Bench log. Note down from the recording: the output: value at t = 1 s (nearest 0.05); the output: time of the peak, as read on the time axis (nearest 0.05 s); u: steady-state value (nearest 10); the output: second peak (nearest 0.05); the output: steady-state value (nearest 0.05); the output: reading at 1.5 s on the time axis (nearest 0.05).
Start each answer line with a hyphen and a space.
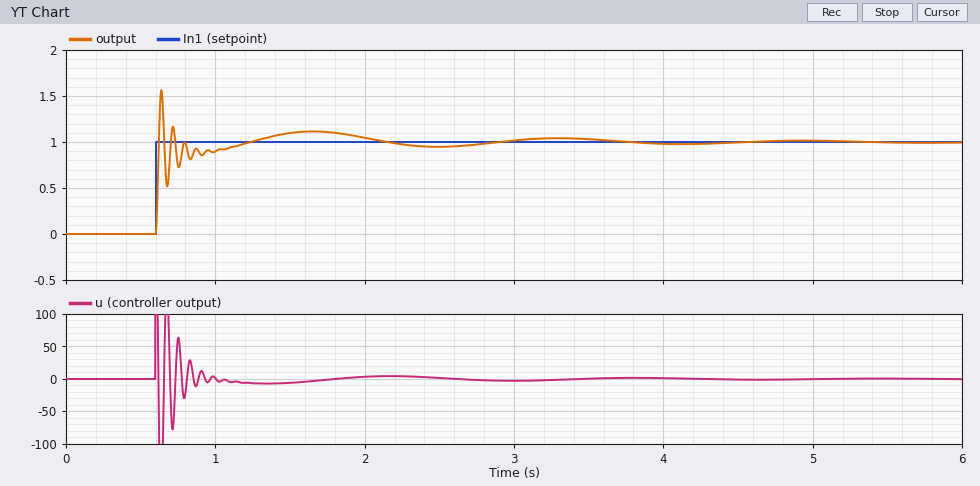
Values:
- 0.90
- 0.65 s
- 0
- 1.15
- 1.00
- 1.10
